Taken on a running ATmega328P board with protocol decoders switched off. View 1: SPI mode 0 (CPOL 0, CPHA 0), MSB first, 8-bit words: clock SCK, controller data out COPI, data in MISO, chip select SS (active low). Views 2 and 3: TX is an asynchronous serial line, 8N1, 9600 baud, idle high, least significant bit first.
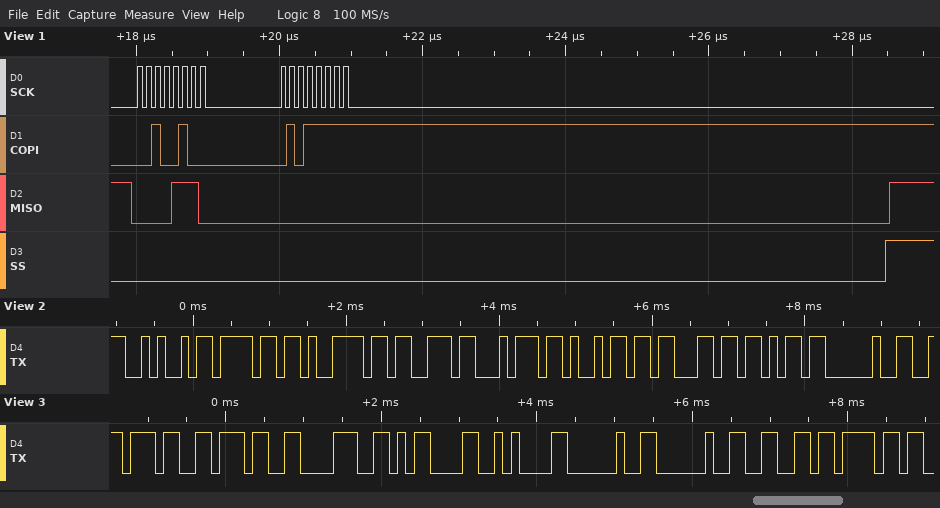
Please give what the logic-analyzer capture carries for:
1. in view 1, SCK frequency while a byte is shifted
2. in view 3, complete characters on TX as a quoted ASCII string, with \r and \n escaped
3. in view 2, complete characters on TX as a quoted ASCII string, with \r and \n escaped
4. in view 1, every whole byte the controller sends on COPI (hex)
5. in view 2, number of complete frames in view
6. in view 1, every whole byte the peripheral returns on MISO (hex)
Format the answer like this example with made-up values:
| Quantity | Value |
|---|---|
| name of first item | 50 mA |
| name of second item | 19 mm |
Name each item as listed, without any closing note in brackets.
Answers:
| Quantity | Value |
|---|---|
| in view 1, SCK frequency while a byte is shifted | 8 MHz |
| in view 3, complete characters on TX as a quoted ASCII string, with \r and \n escaped | "778\r\n  fo" |
| in view 2, complete characters on TX as a quoted ASCII string, with \r and \n escaped | "Joystick " |
| in view 1, every whole byte the controller sends on COPI | 24 5F |
| in view 2, number of complete frames in view | 9 |
| in view 1, every whole byte the peripheral returns on MISO | 0E 00 |
